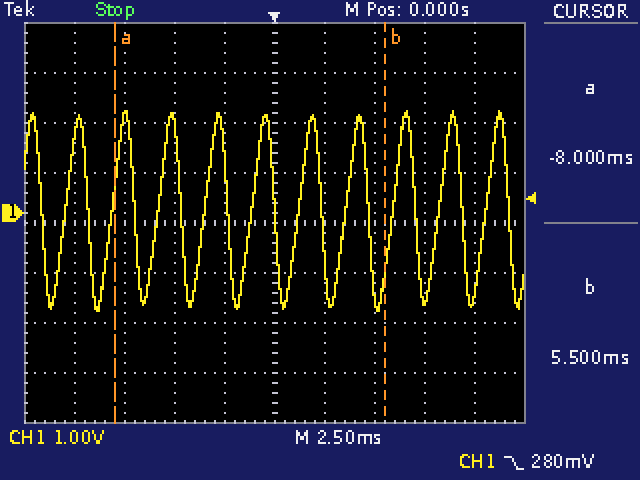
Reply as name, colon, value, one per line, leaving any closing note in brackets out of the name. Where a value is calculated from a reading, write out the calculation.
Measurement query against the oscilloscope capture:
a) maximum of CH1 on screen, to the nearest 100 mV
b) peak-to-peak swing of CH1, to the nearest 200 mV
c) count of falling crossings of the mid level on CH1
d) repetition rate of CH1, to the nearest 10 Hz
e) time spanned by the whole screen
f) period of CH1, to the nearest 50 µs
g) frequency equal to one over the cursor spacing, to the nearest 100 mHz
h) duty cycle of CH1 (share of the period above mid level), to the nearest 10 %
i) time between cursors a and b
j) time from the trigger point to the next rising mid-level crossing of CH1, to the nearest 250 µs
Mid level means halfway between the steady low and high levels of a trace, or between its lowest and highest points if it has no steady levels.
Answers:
maximum of CH1 on screen, to the nearest 100 mV: 2.0 V
peak-to-peak swing of CH1, to the nearest 200 mV: 4.0 V
count of falling crossings of the mid level on CH1: 11
repetition rate of CH1, to the nearest 10 Hz: 1 / 2.35 ms ≈ 426 Hz, so 430 Hz to the nearest 10 Hz
time spanned by the whole screen: 25 ms
period of CH1, to the nearest 50 µs: 2.35 ms
frequency equal to one over the cursor spacing, to the nearest 100 mHz: 1 / 13.50 ms ≈ 74.1 Hz
duty cycle of CH1 (share of the period above mid level), to the nearest 10 %: 50 %
time between cursors a and b: 5.5 ms − (-8 ms) = 13.50 ms
time from the trigger point to the next rising mid-level crossing of CH1, to the nearest 250 µs: 1.25 ms
